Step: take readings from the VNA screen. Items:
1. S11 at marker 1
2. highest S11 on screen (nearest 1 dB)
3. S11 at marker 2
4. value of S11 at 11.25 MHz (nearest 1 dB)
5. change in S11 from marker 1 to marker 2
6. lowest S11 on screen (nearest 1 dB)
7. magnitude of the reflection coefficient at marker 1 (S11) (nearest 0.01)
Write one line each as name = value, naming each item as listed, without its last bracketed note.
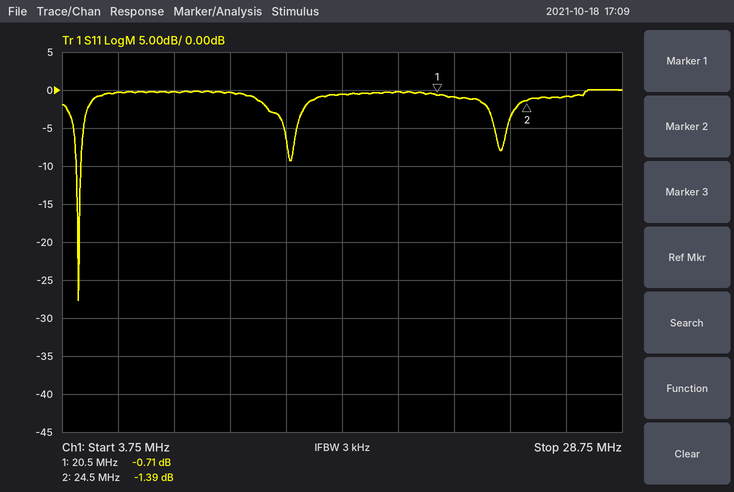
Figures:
S11 at marker 1 = -0.71 dB
highest S11 on screen = 0 dB
S11 at marker 2 = -1.39 dB
value of S11 at 11.25 MHz = 0 dB
change in S11 from marker 1 to marker 2 = -0.68 dB
lowest S11 on screen = -28 dB
magnitude of the reflection coefficient at marker 1 (S11) = 0.92
